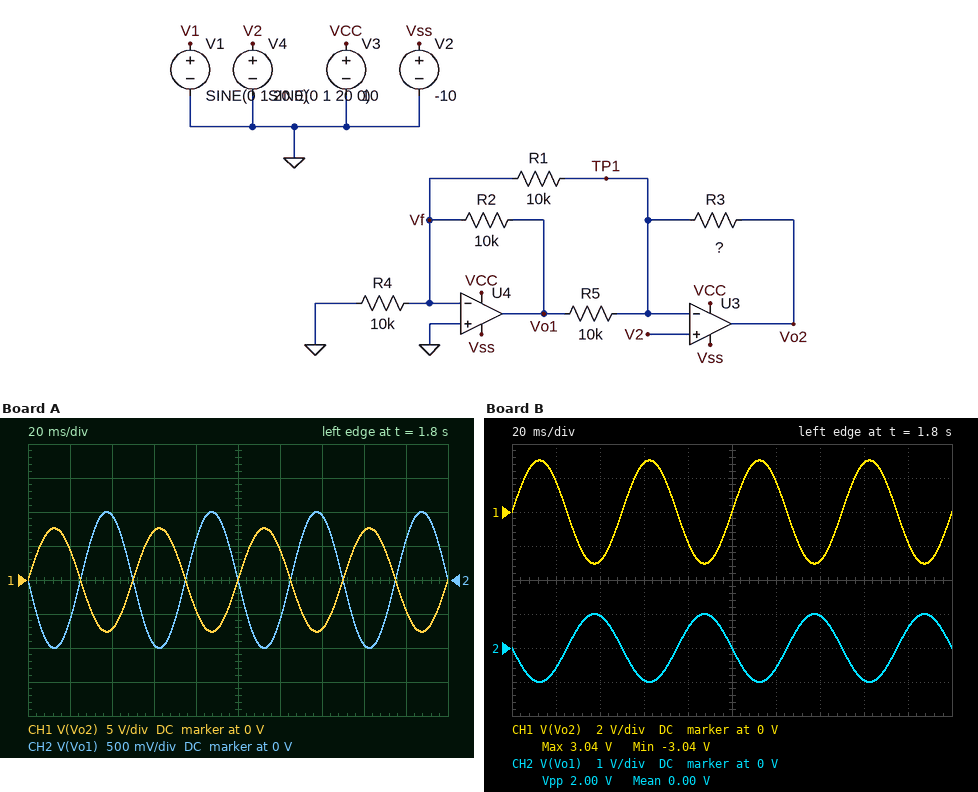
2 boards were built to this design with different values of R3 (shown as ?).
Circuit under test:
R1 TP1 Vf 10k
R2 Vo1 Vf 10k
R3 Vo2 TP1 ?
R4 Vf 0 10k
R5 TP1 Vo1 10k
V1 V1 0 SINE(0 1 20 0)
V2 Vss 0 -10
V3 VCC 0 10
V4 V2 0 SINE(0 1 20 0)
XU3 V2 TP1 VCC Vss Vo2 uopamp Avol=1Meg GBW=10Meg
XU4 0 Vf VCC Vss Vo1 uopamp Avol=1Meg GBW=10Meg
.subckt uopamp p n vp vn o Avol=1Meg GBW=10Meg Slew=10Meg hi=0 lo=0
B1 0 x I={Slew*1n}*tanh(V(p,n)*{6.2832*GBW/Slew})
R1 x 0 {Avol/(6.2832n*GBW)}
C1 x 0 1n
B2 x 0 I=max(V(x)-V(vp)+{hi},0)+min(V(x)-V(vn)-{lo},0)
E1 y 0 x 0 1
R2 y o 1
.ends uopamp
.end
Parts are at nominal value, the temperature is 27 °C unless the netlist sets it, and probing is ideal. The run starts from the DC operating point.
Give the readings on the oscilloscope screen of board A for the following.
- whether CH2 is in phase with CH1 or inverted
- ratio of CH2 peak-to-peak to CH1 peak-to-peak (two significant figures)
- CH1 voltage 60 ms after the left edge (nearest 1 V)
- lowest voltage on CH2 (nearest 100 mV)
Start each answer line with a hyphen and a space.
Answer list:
- inverted
- 0.13
- 7 V
- -1.0 V
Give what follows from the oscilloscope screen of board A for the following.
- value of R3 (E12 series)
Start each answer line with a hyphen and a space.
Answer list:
- 22 kΩ
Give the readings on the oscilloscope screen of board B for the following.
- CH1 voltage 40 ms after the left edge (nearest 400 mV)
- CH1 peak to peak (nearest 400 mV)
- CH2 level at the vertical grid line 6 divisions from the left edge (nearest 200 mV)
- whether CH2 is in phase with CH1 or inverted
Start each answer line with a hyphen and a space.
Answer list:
- -2.8 V
- 6.0 V
- -600 mV
- inverted
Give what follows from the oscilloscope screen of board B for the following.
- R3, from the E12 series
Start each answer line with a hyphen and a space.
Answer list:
- 6.8 kΩ
